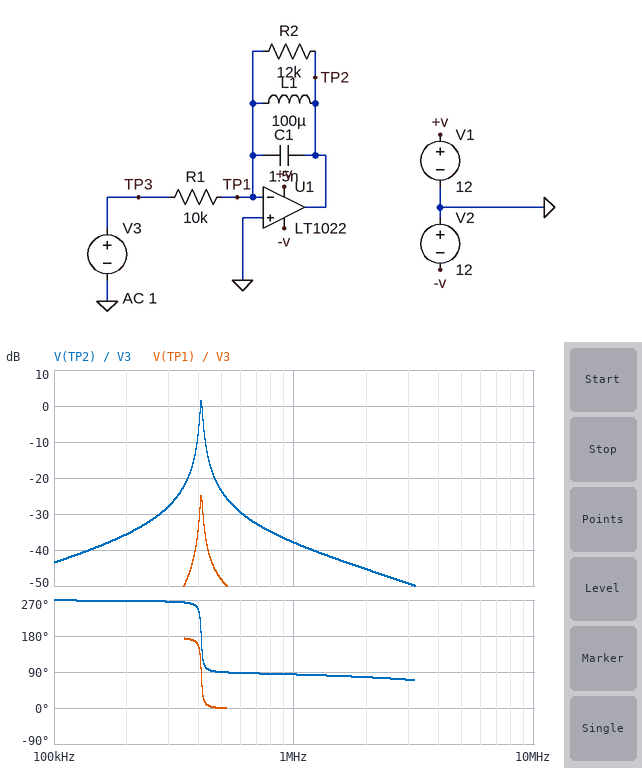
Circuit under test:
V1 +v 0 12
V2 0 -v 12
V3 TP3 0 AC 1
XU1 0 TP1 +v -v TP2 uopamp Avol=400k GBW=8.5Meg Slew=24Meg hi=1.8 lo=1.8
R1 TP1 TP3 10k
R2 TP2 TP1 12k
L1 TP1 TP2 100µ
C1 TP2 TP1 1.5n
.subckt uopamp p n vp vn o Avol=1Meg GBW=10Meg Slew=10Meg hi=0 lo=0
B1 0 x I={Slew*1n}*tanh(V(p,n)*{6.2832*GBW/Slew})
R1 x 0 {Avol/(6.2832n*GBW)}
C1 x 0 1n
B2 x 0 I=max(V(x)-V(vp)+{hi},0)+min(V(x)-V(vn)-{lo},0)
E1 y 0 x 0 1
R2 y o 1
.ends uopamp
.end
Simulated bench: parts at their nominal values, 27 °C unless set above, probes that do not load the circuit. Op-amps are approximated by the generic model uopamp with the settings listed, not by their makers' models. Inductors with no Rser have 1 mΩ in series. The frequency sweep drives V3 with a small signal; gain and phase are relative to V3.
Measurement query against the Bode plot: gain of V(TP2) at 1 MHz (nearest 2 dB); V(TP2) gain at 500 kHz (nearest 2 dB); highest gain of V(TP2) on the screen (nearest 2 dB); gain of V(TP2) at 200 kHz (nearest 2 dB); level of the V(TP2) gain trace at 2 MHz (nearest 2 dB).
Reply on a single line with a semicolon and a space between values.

-38 dB; -24 dB; 2 dB; -36 dB; -46 dB
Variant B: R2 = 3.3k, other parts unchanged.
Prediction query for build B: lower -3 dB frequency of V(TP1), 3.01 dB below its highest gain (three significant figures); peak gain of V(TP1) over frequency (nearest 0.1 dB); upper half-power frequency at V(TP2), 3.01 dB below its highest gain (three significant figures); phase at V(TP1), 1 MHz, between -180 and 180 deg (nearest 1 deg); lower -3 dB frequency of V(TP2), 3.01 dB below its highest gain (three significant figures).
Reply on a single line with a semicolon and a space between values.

396 kHz; -36.0 dB; 427 kHz; -4 deg; 395 kHz
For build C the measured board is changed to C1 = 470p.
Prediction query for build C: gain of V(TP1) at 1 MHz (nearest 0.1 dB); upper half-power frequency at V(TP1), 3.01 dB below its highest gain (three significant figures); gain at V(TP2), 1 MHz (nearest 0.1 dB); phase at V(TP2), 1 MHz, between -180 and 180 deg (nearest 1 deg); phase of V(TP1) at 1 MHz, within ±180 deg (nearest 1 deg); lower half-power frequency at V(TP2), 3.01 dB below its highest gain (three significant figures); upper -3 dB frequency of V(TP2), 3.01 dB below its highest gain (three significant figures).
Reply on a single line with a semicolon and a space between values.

-41.4 dB; 748 kHz; -22.8 dB; 87 deg; -3 deg; 719 kHz; 747 kHz
